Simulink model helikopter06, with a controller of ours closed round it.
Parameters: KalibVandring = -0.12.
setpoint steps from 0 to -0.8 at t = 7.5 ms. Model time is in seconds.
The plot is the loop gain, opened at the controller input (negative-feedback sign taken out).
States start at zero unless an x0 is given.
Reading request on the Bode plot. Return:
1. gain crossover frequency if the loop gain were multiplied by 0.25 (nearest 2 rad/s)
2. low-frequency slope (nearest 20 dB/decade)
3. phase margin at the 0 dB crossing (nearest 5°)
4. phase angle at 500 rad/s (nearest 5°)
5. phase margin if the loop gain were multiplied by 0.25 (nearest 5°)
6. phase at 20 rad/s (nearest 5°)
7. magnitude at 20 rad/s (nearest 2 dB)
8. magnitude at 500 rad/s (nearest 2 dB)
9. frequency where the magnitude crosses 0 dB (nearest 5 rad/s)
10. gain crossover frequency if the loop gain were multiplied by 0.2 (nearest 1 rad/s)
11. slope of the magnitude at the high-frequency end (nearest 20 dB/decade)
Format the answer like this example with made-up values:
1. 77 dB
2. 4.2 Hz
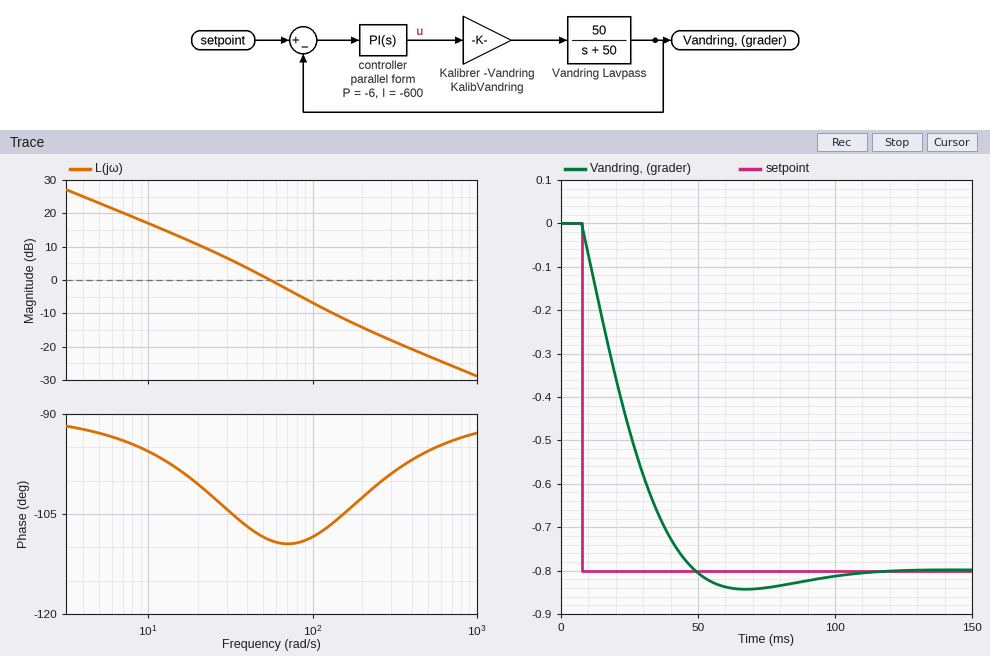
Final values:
1. 18 rad/s
2. -20 dB/decade
3. 70°
4. -95°
5. 80°
6. -100°
7. 10 dB
8. -22 dB
9. 55 rad/s
10. 14 rad/s
11. -20 dB/decade
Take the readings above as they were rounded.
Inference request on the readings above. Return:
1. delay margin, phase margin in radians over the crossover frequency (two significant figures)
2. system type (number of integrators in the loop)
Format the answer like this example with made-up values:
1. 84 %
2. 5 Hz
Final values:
1. 0.022 s
2. 1
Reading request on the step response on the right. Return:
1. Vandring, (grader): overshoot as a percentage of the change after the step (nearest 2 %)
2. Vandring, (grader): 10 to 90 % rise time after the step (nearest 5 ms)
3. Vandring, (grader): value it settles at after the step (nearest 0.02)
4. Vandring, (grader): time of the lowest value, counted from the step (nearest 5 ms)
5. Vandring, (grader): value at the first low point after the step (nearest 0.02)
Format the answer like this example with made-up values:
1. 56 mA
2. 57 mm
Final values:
1. 6 %
2. 30 ms
3. -0.80
4. 60 ms
5. -0.84
